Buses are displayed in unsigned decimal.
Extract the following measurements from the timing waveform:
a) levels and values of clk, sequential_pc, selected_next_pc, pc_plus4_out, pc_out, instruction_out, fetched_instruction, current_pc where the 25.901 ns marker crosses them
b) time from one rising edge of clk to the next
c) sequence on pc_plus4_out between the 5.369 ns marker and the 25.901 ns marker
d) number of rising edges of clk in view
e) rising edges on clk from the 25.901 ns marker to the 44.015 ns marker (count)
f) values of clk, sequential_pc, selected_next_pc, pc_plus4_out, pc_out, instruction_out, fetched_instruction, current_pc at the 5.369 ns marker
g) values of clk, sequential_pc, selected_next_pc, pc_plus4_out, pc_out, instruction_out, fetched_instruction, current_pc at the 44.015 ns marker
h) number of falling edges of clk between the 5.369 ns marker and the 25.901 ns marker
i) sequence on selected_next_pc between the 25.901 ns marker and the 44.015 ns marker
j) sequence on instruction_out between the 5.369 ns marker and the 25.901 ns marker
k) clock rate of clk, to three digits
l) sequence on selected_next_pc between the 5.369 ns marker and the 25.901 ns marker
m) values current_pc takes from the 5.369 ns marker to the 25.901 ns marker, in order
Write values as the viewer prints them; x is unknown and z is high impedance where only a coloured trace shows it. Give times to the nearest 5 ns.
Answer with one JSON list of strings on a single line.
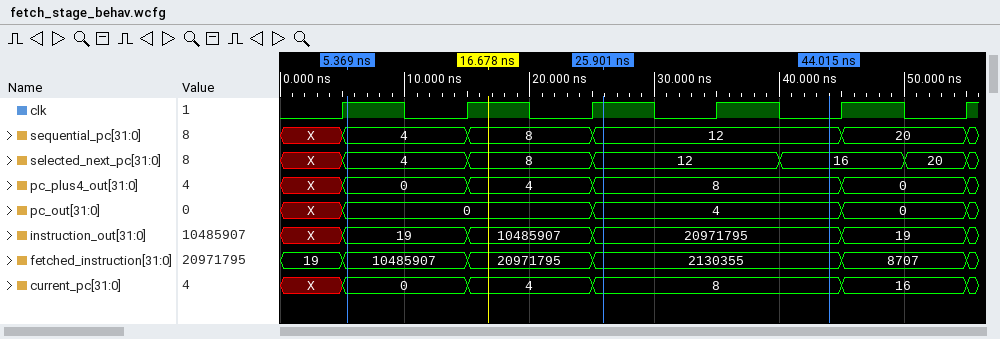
["clk=1, sequential_pc=12, selected_next_pc=12, pc_plus4_out=8, pc_out=4, instruction_out=20971795, fetched_instruction=2130355, current_pc=8", "10 ns", "0, 4, 8", "6", "1", "clk=1, sequential_pc=4, selected_next_pc=4, pc_plus4_out=0, pc_out=0, instruction_out=19, fetched_instruction=10485907, current_pc=0", "clk=0, sequential_pc=12, selected_next_pc=16, pc_plus4_out=8, pc_out=4, instruction_out=20971795, fetched_instruction=2130355, current_pc=8", "2", "12, 16", "19, 10485907, 20971795", "100 MHz", "4, 8, 12", "0, 4, 8"]
